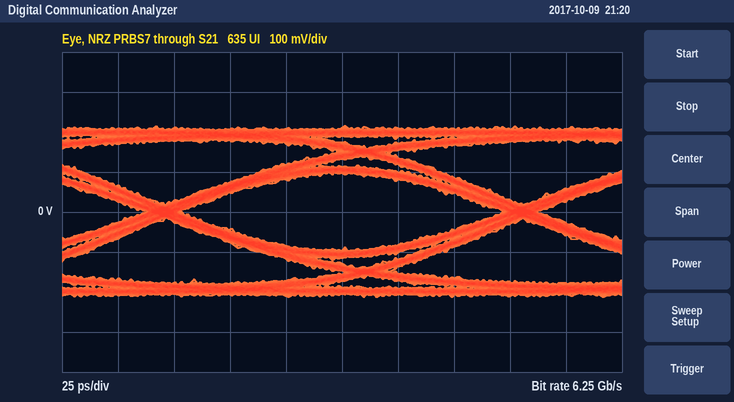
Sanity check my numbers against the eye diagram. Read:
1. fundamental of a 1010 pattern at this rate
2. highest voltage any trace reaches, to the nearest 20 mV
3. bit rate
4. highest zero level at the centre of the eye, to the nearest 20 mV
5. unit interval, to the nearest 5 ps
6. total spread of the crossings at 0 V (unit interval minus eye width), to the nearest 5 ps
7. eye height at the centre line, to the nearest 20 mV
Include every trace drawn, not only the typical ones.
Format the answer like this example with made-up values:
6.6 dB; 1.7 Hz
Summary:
3.125 GHz; 220 mV; 6.25 Gb/s; -100 mV; 160 ps; 15 ps; 200 mV
